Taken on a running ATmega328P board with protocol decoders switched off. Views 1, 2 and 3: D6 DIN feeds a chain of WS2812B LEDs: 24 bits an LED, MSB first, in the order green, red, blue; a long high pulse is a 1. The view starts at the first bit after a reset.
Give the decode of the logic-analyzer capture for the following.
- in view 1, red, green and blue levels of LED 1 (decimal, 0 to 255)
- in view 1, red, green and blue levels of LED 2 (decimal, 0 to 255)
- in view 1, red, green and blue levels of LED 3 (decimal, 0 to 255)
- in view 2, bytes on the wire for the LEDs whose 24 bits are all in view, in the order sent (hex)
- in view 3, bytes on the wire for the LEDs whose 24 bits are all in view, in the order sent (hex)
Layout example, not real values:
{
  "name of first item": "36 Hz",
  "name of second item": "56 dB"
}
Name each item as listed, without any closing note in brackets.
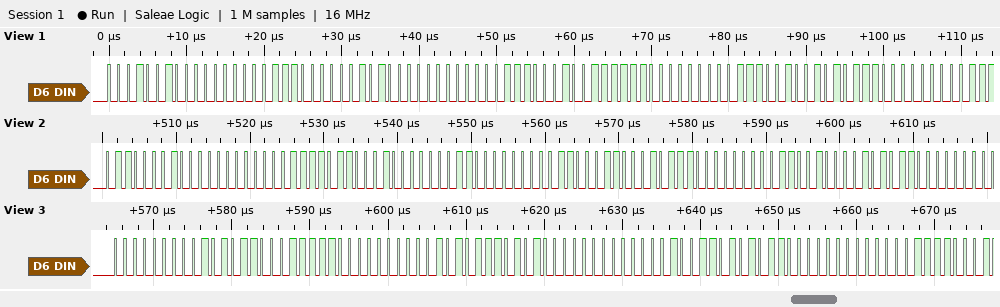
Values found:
{
  "in view 1, red, green and blue levels of LED 1": "0, 18, 112",
  "in view 1, red, green and blue levels of LED 2": "0, 40, 113",
  "in view 1, red, green and blue levels of LED 3": "0, 63, 114",
  "in view 2, bytes on the wire for the LEDs whose 24 bits are all in view, in the order sent": "61 00 0F 62 03 00 63 17 00 64 2B 00",
  "in view 3, bytes on the wire for the LEDs whose 24 bits are all in view, in the order sent": "00 56 3E 00 57 50 00 4D 58"
}
